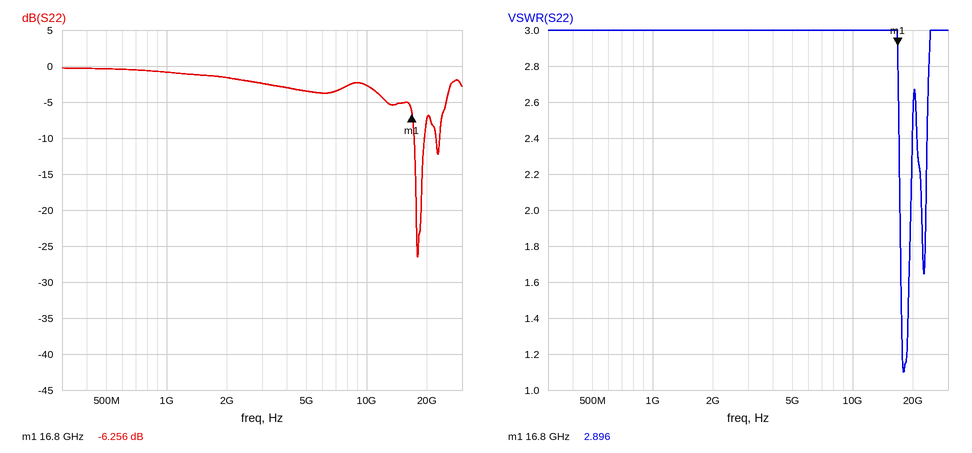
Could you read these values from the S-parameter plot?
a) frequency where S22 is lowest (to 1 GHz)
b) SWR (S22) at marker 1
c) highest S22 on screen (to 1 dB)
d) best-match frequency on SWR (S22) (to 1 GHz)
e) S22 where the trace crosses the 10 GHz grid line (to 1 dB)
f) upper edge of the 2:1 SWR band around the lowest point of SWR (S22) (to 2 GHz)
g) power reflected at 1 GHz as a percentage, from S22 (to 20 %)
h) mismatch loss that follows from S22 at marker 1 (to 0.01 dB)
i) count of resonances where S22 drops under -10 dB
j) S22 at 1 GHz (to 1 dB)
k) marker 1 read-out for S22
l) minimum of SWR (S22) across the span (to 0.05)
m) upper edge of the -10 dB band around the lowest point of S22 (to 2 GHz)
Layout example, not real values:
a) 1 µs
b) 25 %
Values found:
a) 18 GHz
b) 2.896
c) 0 dB
d) 18 GHz
e) -3 dB
f) 20 GHz
g) 80 %
h) 1.17 dB
i) 2
j) -1 dB
k) -6.256 dB
l) 1.10
m) 20 GHz
